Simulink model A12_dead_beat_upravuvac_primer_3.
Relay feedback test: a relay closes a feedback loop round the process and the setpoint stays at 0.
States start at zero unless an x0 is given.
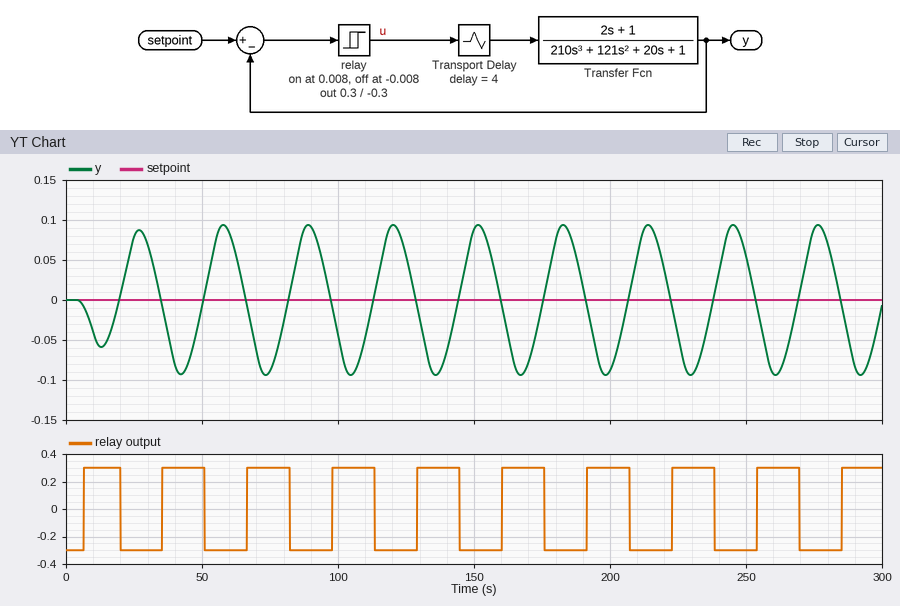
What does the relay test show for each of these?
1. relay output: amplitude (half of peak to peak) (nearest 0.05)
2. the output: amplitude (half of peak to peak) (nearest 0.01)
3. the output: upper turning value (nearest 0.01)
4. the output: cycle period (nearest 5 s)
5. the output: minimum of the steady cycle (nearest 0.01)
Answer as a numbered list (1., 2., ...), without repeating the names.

1. 0.30
2. 0.09
3. 0.09
4. 30 s
5. -0.09
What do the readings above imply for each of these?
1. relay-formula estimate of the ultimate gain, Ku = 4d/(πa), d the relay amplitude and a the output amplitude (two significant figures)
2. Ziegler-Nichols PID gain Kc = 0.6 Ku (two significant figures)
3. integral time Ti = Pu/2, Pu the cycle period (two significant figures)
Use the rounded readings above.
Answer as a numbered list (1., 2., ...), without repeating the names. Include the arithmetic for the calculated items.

1. 4 × 0.3 / (π × 0.09) = 4.2
2. 0.6 × 4.2 = 2.5
3. 30 / 2 = 15 s
